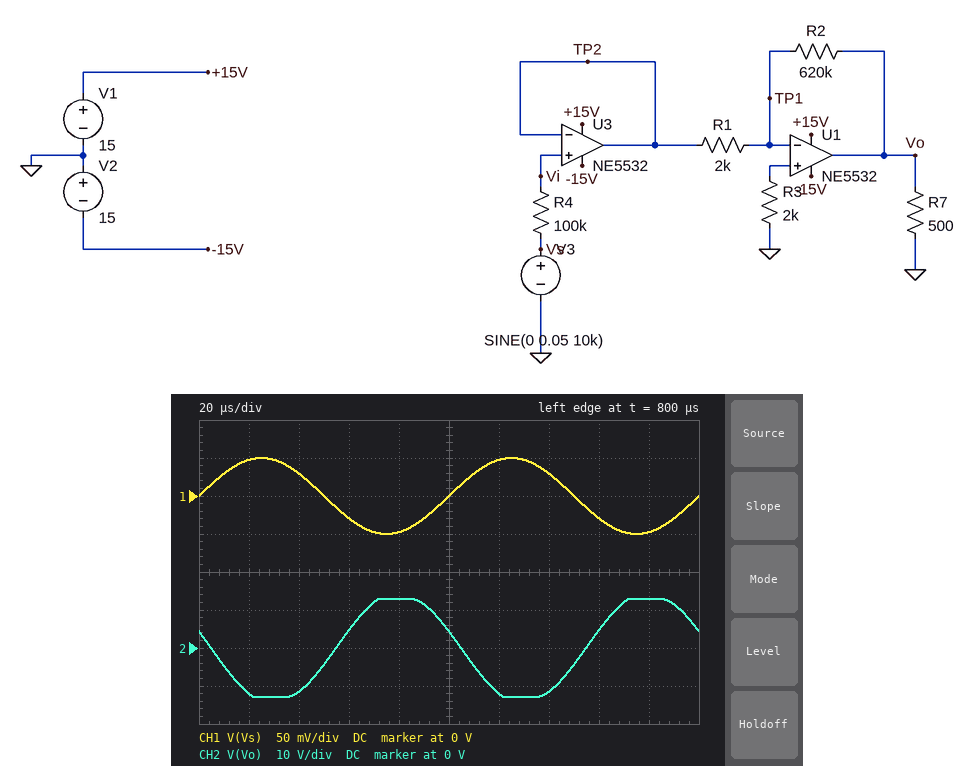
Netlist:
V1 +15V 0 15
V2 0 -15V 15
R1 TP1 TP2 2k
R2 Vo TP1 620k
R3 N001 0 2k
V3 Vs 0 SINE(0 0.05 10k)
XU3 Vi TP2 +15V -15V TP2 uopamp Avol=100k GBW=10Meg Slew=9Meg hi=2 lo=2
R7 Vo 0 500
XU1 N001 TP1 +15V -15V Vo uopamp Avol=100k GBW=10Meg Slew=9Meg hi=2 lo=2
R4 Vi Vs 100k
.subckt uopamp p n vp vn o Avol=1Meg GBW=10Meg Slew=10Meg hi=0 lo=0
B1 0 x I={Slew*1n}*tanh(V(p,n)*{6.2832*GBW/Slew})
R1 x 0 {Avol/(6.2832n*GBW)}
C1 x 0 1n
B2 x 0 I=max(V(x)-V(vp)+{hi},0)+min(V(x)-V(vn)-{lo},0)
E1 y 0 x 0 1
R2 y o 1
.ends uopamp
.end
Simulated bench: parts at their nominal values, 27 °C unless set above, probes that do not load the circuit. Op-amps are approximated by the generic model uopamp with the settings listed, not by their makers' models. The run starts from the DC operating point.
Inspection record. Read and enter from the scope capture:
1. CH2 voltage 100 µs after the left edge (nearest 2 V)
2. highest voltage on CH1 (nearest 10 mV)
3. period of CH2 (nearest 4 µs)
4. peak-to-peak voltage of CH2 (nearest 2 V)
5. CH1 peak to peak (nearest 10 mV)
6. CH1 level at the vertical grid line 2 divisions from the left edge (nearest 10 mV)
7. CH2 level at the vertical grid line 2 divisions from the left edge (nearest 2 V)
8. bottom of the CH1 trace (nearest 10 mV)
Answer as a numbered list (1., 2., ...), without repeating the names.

1. 4 V
2. 50 mV
3. 100 µs
4. 26 V
5. 100 mV
6. 30 mV
7. -12 V
8. -50 mV
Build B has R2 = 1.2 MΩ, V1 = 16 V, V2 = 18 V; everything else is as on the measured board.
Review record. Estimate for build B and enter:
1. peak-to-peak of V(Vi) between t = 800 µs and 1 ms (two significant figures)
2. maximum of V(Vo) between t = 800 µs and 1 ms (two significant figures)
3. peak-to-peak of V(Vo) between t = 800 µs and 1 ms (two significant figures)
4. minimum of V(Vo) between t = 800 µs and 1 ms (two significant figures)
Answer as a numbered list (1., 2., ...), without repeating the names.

1. 100 mV
2. 14 V
3. 30 V
4. -16 V
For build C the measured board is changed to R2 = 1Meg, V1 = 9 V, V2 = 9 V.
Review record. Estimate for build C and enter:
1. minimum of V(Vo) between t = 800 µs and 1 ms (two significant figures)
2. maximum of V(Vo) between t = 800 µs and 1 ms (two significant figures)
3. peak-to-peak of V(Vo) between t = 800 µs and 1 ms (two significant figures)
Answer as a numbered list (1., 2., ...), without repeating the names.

1. -7.0 V
2. 7.0 V
3. 14 V
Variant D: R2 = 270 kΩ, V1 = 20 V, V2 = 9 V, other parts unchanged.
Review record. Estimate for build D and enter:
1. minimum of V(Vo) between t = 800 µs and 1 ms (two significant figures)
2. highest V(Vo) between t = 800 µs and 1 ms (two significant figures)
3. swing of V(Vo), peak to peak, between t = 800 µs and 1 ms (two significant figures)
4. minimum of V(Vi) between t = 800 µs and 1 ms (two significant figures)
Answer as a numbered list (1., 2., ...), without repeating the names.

1. -6.7 V
2. 6.7 V
3. 13 V
4. -50 mV
